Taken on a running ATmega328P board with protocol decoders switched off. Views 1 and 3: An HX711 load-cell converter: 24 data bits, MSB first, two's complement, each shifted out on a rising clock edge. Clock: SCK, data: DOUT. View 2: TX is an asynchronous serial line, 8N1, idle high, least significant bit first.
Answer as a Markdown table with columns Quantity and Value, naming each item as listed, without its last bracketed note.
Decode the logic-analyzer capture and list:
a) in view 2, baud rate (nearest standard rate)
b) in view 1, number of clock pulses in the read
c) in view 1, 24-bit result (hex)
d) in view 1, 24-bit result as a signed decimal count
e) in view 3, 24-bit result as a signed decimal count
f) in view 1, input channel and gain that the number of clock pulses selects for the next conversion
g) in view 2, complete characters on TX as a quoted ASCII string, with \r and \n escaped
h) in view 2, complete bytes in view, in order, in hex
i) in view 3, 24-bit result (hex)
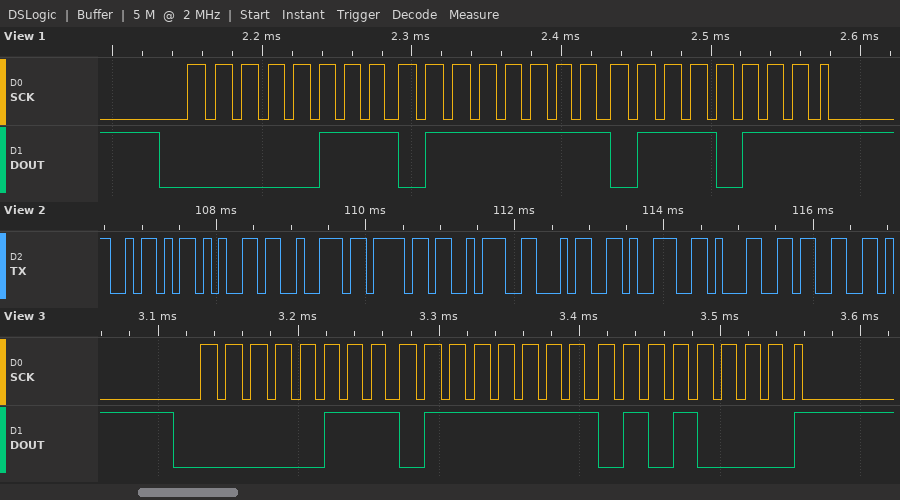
| Quantity | Value |
|---|---|
| in view 2, baud rate | 9600 baud |
| in view 1, number of clock pulses in the read | 25 |
| in view 1, 24-bit result | 0x077F77 |
| in view 1, 24-bit result as a signed decimal count | 491383 |
| in view 3, 24-bit result as a signed decimal count | 491344 |
| in view 1, input channel and gain that the number of clock pulses selects for the next conversion | channel A, gain 128 |
| in view 2, complete characters on TX as a quoted ASCII string, with \r and \n escaped | "Zero:4913" |
| in view 2, complete bytes in view, in order, in hex | 5A 65 72 6F 3A 34 39 31 33 |
| in view 3, 24-bit result | 0x077F50 |
